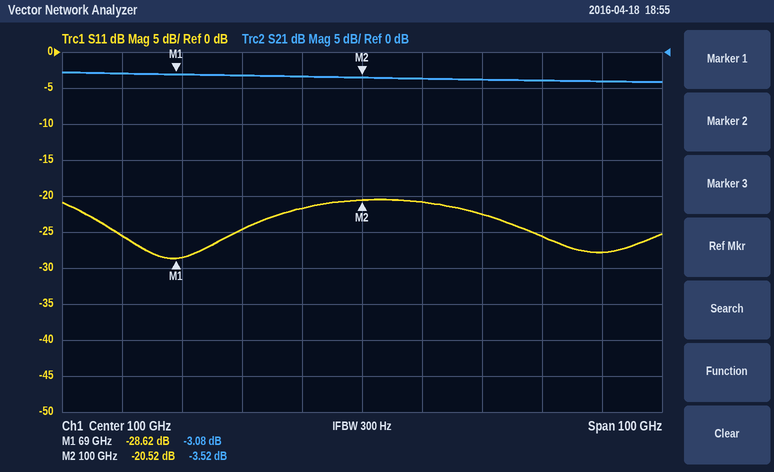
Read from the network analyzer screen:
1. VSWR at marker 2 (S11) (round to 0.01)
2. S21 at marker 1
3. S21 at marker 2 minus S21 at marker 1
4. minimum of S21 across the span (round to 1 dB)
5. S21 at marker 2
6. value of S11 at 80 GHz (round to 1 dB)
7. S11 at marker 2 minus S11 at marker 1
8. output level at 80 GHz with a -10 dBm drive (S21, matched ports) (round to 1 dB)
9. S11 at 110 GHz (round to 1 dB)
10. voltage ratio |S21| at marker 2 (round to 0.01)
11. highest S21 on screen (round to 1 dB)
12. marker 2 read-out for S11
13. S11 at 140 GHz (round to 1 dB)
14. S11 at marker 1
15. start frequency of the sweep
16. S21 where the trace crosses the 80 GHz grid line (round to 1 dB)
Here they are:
1.21
-3.08 dB
-0.44 dB
-4 dB
-3.52 dB
-25 dB
8.10 dB
-13 dBm
-21 dB
0.67
-3 dB
-20.52 dB
-28 dB
-28.62 dB
50 GHz
-3 dB
